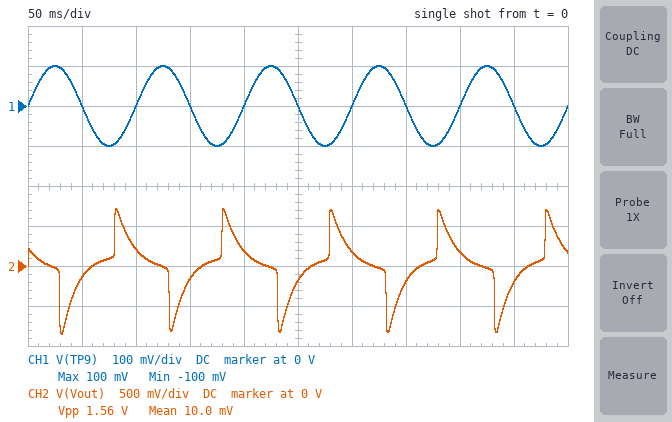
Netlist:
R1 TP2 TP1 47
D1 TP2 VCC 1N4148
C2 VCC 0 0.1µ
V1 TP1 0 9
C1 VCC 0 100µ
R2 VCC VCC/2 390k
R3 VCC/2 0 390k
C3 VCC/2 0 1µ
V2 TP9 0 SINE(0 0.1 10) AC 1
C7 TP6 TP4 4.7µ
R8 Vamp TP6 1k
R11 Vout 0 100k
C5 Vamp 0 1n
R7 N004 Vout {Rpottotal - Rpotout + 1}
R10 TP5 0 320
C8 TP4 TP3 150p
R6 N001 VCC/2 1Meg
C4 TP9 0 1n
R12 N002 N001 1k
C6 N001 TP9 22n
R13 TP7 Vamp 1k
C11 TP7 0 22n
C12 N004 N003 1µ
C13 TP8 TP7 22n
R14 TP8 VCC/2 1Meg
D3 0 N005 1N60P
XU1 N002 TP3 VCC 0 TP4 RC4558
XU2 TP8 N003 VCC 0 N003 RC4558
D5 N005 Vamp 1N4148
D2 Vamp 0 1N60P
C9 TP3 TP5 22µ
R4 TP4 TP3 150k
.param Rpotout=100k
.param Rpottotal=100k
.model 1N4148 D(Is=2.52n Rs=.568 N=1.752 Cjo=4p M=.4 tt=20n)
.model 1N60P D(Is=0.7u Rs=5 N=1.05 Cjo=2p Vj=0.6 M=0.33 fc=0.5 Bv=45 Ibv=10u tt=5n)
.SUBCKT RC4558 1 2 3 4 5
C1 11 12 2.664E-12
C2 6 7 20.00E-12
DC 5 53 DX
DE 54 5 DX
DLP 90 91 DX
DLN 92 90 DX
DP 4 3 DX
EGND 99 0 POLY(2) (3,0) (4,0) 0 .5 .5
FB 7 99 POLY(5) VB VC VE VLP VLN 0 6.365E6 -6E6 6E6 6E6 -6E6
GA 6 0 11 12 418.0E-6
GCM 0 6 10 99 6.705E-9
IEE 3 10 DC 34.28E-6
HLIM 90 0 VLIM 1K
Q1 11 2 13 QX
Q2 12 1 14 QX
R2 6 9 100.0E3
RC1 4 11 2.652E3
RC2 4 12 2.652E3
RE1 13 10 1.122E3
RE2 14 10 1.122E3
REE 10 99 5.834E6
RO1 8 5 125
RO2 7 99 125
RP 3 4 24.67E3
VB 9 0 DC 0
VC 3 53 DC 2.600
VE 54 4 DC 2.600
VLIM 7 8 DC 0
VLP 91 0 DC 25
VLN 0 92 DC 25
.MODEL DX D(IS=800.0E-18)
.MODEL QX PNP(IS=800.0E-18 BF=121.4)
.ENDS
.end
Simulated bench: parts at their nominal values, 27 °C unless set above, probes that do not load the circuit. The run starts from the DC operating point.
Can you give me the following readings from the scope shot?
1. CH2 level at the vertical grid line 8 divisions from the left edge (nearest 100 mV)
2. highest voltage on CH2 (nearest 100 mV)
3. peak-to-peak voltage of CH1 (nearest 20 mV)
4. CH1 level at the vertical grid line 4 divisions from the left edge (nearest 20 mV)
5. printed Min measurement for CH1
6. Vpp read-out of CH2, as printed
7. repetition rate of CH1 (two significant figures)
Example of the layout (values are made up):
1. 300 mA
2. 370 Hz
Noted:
1. 200 mV
2. 700 mV
3. 200 mV
4. 0 V
5. -100 mV
6. 1.56 V
7. 10 Hz
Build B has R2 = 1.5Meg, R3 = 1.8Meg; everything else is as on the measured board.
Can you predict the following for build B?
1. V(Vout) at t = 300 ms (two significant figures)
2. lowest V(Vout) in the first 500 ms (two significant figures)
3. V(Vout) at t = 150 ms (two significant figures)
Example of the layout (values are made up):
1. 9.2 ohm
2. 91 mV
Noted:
1. 130 mV
2. -840 mV
3. -220 mV
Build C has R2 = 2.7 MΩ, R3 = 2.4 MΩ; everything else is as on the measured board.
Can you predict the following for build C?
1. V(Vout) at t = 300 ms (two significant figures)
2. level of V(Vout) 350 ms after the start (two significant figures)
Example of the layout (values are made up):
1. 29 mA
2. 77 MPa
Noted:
1. 170 mV
2. -200 mV
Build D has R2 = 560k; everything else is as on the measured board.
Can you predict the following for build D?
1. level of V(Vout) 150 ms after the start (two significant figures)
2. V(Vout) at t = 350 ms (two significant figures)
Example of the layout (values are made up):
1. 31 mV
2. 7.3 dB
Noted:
1. -97 mV
2. -91 mV
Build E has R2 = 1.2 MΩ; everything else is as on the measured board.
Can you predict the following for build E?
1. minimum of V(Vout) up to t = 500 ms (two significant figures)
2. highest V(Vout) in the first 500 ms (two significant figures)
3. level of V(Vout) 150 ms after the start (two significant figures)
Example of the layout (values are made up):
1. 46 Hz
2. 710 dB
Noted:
1. -410 mV
2. 660 mV
3. -39 mV
